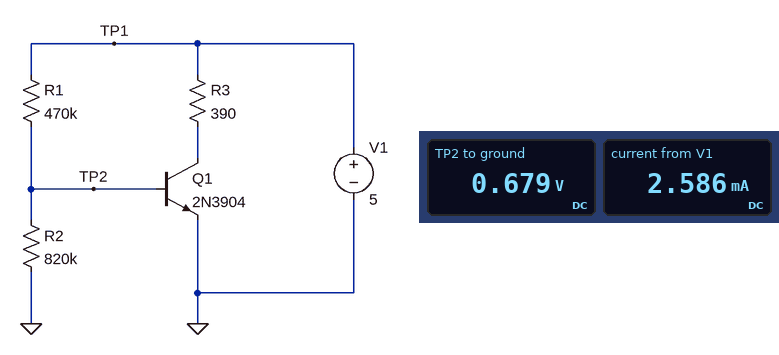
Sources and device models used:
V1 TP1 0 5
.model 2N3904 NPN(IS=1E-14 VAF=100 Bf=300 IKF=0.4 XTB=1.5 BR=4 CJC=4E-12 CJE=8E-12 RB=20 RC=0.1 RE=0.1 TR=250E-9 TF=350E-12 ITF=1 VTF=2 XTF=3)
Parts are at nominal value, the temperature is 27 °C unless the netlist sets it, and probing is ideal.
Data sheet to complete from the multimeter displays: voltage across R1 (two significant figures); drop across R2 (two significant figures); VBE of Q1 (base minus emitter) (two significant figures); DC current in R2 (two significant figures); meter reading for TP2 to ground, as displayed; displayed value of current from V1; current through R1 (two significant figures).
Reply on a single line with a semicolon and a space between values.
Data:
4.3 V; 680 mV; 680 mV; 830 nA; 0.679 V; 2.586 mA; 9.2 µA
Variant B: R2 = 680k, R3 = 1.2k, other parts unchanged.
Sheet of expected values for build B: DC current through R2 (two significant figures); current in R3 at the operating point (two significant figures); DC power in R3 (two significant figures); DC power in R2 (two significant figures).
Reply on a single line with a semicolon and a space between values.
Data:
1.0 µA; 2.5 mA; 7.4 mW; 680 nW
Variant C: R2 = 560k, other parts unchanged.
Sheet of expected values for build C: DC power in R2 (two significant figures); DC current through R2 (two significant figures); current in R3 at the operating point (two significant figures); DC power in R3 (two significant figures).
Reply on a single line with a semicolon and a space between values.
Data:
820 nW; 1.2 µA; 2.5 mA; 2.4 mW
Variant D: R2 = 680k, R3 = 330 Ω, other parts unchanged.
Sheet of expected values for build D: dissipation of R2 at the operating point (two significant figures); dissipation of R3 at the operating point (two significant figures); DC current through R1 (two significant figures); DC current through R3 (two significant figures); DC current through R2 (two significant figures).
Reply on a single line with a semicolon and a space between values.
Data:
680 nW; 2.1 mW; 9.2 µA; 2.5 mA; 1.0 µA
